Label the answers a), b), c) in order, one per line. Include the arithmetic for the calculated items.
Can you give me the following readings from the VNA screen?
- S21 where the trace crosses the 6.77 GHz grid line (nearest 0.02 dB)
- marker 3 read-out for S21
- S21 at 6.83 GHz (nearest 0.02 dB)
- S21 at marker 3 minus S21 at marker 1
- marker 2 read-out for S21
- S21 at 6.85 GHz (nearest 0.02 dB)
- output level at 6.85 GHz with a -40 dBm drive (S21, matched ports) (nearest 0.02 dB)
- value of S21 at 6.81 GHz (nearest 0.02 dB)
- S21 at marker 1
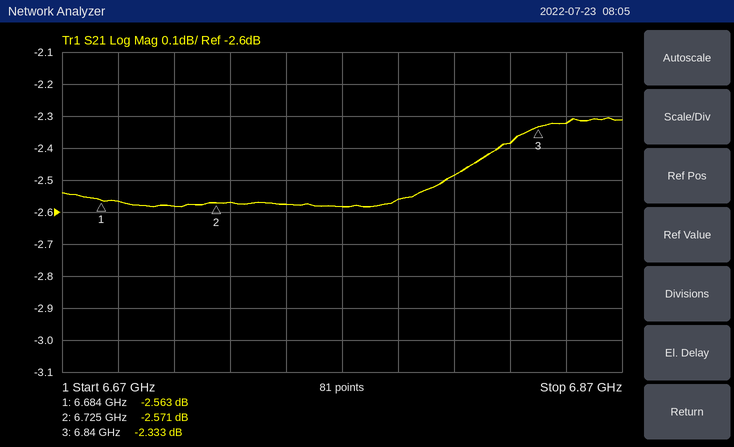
a) -2.58 dB
b) -2.333 dB
c) -2.38 dB
d) -2.333 − (-2.563) = 0.230 dB
e) -2.571 dB
f) -2.32 dB
g) -40 dBm + (-2.32 dB) = -42.32 dBm
h) -2.48 dB
i) -2.563 dB
